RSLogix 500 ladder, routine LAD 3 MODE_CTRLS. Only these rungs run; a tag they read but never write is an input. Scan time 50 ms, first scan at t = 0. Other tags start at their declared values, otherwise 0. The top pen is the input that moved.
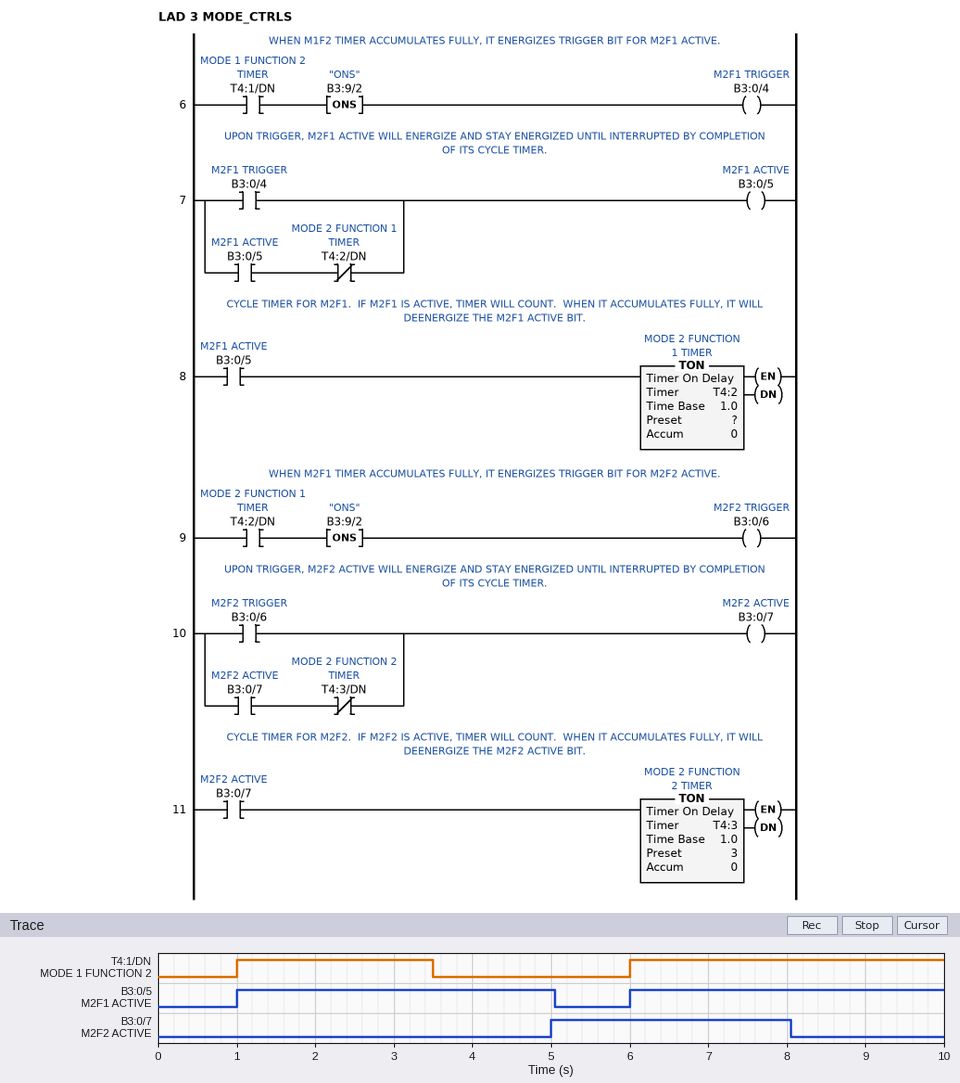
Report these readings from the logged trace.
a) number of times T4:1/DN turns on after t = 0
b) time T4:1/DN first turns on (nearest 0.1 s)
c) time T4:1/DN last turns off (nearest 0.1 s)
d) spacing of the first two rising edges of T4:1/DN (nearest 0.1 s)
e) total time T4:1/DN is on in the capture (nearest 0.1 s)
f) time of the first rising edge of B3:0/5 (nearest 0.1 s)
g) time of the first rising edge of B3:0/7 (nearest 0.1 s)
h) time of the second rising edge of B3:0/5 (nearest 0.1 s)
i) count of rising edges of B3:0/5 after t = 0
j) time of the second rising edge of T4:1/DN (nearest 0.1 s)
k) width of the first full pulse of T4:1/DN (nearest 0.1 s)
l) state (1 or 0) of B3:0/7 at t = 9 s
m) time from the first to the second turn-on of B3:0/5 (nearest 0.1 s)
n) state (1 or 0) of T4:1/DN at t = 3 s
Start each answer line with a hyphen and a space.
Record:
- 2
- 1.0 s
- 3.5 s
- 5.0 s
- 6.5 s
- 1.0 s
- 5.0 s
- 6.0 s
- 2
- 6.0 s
- 2.5 s
- 0
- 5.0 s
- 1
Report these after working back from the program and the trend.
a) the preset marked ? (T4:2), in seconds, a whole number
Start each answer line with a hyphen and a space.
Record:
- 4 s
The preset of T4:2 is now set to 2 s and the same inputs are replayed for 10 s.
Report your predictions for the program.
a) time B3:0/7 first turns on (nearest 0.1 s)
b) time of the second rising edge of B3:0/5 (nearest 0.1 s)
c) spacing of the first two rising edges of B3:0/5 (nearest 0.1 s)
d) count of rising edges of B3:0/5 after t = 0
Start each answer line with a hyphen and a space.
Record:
- 5.1 s
- 3.1 s
- 2.1 s
- 4
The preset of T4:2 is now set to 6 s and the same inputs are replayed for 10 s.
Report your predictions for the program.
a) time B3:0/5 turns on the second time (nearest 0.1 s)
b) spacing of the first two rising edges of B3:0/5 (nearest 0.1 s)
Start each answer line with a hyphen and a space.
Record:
- 7.1 s
- 6.1 s
